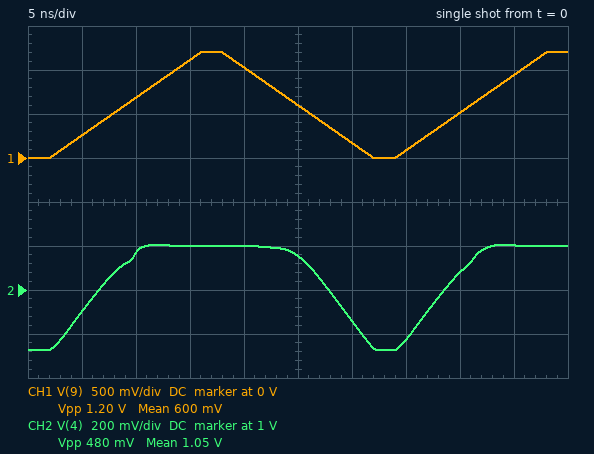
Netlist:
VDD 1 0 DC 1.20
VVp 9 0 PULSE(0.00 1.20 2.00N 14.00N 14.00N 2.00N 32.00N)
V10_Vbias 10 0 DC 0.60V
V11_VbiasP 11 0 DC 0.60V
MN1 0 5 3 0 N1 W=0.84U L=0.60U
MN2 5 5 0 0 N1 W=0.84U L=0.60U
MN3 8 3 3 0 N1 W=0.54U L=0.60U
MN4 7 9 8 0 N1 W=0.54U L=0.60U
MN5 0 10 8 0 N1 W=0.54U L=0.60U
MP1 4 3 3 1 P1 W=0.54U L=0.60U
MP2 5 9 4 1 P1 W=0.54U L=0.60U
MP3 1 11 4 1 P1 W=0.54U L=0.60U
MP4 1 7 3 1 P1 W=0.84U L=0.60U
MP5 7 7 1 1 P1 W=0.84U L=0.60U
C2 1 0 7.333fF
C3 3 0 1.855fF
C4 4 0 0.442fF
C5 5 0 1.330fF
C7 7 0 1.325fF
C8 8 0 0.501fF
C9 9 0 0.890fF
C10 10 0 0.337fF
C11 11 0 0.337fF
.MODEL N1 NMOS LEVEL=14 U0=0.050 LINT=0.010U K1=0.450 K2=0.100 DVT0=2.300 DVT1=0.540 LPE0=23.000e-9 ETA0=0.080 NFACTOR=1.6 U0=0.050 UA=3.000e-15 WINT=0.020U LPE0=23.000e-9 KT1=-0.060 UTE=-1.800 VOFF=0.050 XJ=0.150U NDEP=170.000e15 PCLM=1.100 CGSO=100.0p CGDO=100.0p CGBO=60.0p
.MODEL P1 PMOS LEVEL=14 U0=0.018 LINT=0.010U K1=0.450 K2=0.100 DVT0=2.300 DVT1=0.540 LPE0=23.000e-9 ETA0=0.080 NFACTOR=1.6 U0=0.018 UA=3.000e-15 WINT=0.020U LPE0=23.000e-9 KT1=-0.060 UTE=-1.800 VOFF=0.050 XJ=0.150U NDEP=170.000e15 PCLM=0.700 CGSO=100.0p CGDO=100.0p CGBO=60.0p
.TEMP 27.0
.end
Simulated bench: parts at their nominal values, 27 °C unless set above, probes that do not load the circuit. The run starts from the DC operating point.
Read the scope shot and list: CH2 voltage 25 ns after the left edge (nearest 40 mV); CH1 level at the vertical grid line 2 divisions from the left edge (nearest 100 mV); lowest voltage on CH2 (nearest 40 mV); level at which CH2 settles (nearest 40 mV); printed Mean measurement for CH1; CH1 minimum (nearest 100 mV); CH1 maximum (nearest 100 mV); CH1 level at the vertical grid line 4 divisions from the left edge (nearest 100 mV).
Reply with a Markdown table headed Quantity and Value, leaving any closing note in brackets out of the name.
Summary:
| Quantity | Value |
|---|---|
| CH2 voltage 25 ns after the left edge | 1.16 V |
| CH1 level at the vertical grid line 2 divisions from the left edge | 700 mV |
| lowest voltage on CH2 | 720 mV |
| level at which CH2 settles | 1.20 V |
| printed Mean measurement for CH1 | 600 mV |
| CH1 minimum | 0 V |
| CH1 maximum | 1.2 V |
| CH1 level at the vertical grid line 4 divisions from the left edge | 1.0 V |
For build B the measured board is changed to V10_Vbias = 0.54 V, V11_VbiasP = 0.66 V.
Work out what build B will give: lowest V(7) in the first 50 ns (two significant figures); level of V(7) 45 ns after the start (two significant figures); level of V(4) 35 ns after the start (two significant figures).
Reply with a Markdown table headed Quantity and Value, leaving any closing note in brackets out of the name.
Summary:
| Quantity | Value |
|---|---|
| lowest V(7) in the first 50 ns | 650 mV |
| level of V(7) 45 ns after the start | 660 mV |
| level of V(4) 35 ns after the start | 720 mV |
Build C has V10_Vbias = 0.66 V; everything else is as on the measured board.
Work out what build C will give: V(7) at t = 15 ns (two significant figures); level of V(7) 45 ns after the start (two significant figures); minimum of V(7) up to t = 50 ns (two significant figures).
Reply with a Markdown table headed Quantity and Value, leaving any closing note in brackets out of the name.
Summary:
| Quantity | Value |
|---|---|
| V(7) at t = 15 ns | 550 mV |
| level of V(7) 45 ns after the start | 560 mV |
| minimum of V(7) up to t = 50 ns | 540 mV |
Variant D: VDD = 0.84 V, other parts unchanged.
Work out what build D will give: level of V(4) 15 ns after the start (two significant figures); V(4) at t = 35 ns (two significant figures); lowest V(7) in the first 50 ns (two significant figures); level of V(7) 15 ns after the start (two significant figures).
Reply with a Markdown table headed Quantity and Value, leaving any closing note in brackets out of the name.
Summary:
| Quantity | Value |
|---|---|
| level of V(4) 15 ns after the start | 480 mV |
| V(4) at t = 35 ns | 410 mV |
| lowest V(7) in the first 50 ns | 230 mV |
| level of V(7) 15 ns after the start | 240 mV |
